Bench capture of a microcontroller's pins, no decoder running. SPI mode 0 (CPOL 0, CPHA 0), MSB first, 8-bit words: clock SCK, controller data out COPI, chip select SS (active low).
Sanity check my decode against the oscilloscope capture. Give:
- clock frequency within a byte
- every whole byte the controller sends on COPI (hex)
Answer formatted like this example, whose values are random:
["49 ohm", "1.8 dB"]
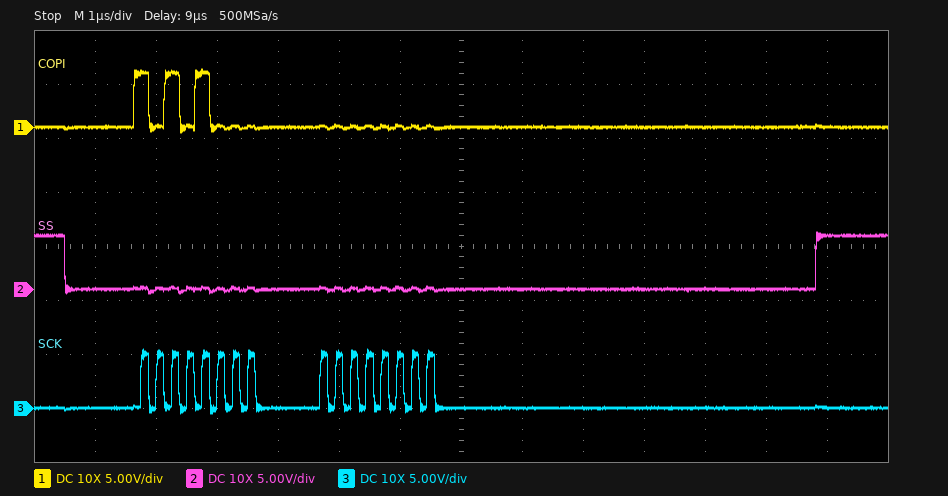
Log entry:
["4 MHz", "A8 00"]
